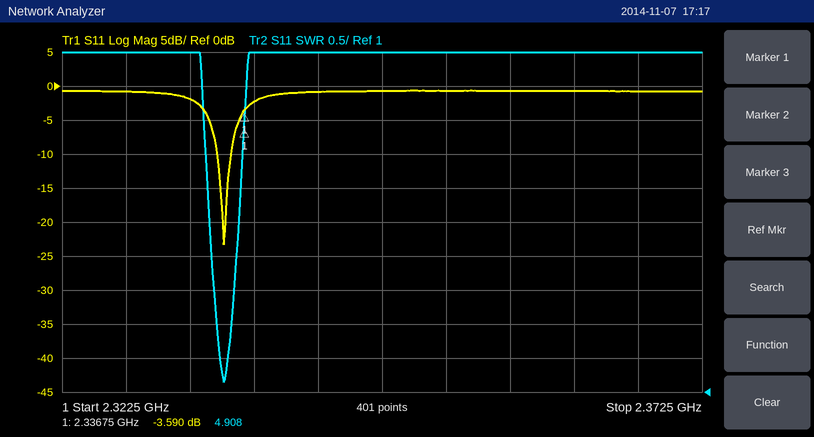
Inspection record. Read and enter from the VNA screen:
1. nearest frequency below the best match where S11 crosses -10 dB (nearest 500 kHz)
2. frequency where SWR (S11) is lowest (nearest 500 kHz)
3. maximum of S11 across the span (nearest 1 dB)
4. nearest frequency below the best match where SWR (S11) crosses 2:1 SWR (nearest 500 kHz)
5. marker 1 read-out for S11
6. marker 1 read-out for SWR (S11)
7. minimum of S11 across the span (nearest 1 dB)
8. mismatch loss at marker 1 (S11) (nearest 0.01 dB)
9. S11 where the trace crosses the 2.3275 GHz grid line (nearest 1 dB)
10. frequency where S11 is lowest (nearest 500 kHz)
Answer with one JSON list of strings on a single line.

["2.3345 GHz", "2.3350 GHz", "-1 dB", "2.3345 GHz", "-3.590 dB", "4.908", "-23 dB", "2.50 dB", "-1 dB", "2.3350 GHz"]
